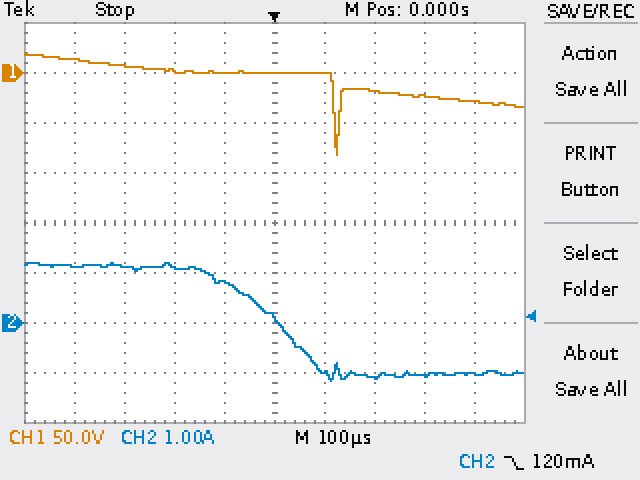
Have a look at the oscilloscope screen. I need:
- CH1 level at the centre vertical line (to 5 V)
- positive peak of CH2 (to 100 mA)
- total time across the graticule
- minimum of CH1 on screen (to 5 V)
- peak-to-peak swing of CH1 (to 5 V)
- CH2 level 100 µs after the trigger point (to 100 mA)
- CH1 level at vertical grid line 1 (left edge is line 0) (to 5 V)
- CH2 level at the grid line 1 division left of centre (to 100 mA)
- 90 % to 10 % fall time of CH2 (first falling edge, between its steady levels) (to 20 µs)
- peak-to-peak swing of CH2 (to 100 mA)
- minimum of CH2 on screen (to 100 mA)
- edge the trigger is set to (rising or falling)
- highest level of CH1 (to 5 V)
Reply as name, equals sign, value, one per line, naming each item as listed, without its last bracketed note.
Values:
CH1 level at the centre vertical line = 0 V
positive peak of CH2 = 1.2 A
total time across the graticule = 1 ms
minimum of CH1 on screen = -80 V
peak-to-peak swing of CH1 = 100 V
CH2 level 100 µs after the trigger point = -1.0 A
CH1 level at vertical grid line 1 (left edge is line 0) = 15 V
CH2 level at the grid line 1 division left of centre = 800 mA
90 % to 10 % fall time of CH2 (first falling edge, between its steady levels) = 200 µs
peak-to-peak swing of CH2 = 2.4 A
minimum of CH2 on screen = -1.2 A
edge the trigger is set to = falling
highest level of CH1 = 20 V
